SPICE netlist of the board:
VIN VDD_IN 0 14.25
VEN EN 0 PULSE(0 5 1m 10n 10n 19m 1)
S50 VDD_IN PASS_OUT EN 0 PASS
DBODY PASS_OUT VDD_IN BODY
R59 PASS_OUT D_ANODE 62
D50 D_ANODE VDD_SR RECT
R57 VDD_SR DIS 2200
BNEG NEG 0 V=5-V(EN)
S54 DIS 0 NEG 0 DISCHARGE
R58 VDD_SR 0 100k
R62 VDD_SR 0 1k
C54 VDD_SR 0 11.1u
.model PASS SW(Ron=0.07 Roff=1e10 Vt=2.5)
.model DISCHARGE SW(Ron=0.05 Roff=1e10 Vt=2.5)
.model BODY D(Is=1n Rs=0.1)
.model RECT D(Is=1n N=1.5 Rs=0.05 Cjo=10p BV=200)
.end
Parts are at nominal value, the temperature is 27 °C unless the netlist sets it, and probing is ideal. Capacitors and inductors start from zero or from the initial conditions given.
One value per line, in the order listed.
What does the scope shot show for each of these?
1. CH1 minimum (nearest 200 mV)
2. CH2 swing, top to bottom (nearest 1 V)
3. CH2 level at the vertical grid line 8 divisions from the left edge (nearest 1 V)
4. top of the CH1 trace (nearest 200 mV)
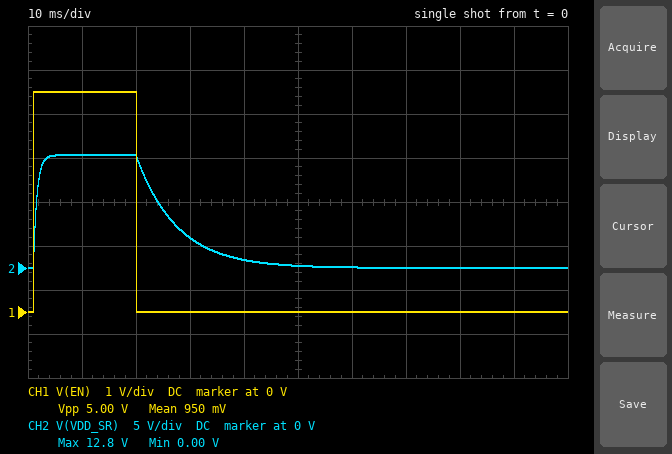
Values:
0 V
13 V
0 V
5.0 V
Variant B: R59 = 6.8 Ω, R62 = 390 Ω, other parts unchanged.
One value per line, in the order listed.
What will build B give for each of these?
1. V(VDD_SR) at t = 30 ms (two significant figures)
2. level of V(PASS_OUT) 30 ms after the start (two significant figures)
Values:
870 mV
920 mV
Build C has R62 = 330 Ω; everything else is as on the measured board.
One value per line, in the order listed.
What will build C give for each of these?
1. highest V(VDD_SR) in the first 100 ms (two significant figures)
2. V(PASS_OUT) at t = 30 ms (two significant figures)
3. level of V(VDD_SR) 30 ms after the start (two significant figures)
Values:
11 V
540 mV
490 mV
